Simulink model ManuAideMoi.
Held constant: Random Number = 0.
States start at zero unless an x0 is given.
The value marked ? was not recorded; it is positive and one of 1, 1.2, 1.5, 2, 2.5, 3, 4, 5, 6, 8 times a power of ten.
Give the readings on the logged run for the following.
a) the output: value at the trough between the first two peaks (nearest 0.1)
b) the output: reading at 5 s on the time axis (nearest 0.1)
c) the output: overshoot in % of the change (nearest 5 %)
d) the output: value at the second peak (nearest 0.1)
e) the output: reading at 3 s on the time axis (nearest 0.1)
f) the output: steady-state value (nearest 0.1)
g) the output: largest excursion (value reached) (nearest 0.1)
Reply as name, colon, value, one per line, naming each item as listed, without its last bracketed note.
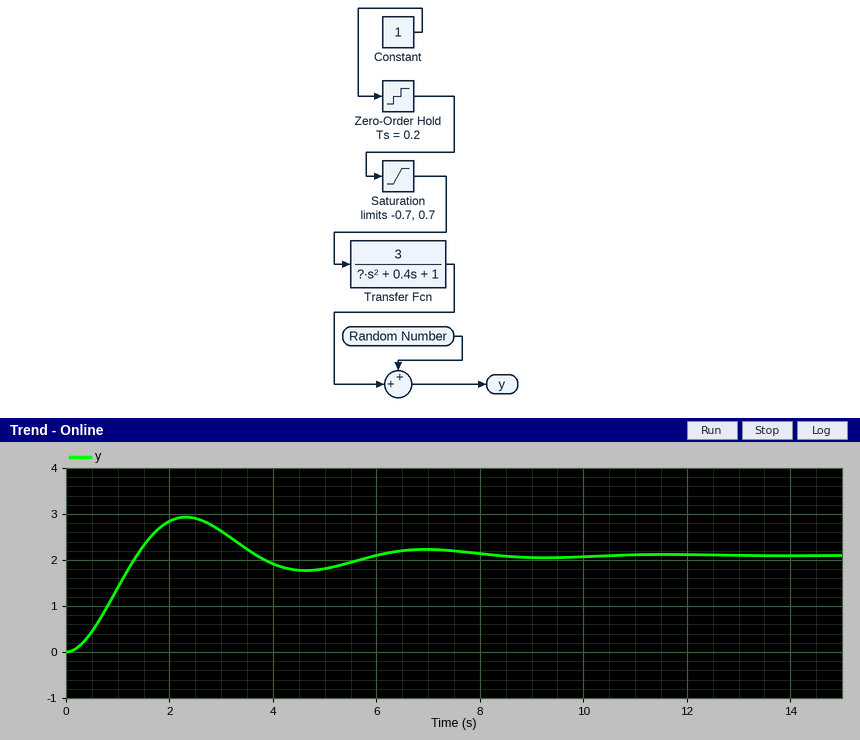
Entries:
the output: value at the trough between the first two peaks: 1.8
the output: reading at 5 s on the time axis: 1.8
the output: overshoot in % of the change: 40 %
the output: value at the second peak: 2.2
the output: reading at 3 s on the time axis: 2.6
the output: steady-state value: 2.1
the output: largest excursion (value reached): 2.9
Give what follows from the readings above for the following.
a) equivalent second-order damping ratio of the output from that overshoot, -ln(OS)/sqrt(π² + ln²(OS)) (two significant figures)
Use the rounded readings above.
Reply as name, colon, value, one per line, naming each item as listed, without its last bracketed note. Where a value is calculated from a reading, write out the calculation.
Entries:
equivalent second-order damping ratio of the output from that overshoot, -ln(OS)/sqrt(π² + ln²(OS)): ln(0.4) = -0.916; 0.916 / sqrt(9.870 + 0.840) = 0.28
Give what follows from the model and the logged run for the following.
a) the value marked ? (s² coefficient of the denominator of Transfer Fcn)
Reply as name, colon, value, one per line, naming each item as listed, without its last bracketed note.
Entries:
the value marked ?: 0.5
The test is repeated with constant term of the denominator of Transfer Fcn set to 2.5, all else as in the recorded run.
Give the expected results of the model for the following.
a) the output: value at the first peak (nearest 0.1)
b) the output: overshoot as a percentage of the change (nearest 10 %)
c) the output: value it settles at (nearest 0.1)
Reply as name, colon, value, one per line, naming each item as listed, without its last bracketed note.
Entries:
the output: value at the first peak: 1.3
the output: overshoot as a percentage of the change: 60 %
the output: value it settles at: 0.8
